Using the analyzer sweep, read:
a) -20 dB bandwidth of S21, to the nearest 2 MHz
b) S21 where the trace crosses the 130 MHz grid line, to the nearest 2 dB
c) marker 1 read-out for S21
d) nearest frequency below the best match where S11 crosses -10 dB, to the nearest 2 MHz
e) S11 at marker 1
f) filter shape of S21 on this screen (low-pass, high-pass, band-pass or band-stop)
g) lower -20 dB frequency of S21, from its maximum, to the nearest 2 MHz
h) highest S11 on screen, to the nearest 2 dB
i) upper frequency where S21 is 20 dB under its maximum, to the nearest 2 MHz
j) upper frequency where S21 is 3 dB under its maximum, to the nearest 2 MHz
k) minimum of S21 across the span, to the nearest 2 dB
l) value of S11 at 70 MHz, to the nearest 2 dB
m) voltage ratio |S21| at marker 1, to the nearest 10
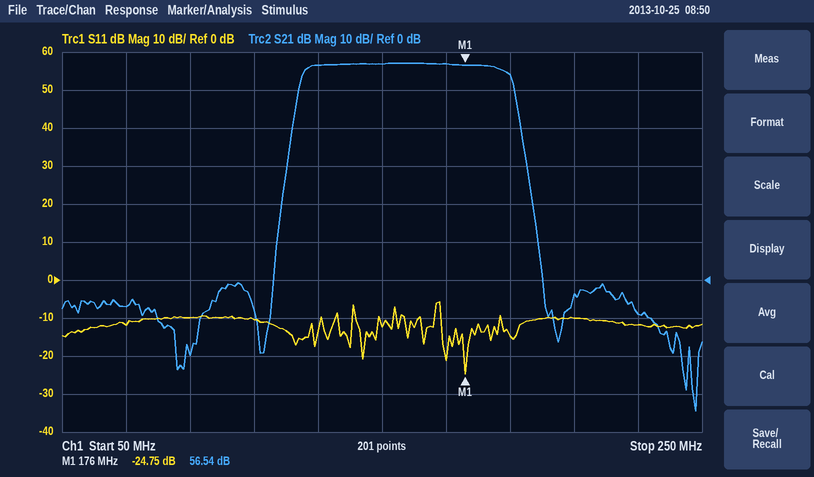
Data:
72 MHz
56 dB
56.54 dB
168 MHz
-24.75 dB
band-pass
122 MHz
-6 dB
194 MHz
190 MHz
-34 dB
-12 dB
670
